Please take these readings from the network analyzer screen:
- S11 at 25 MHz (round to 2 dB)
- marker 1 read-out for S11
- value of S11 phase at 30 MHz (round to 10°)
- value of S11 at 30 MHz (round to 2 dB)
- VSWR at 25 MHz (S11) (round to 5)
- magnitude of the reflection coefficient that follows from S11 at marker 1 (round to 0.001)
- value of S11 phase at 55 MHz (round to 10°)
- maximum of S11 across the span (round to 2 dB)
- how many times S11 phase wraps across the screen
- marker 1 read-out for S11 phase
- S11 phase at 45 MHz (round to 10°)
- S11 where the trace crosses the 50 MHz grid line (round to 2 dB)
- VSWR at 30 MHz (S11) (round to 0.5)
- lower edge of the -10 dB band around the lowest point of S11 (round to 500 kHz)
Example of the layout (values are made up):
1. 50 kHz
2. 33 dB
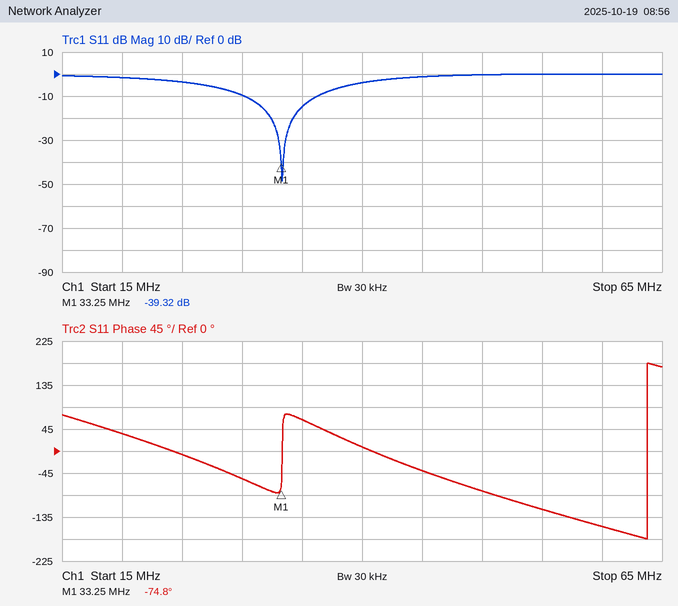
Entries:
1. -4 dB
2. -39.32 dB
3. -60°
4. -10 dB
5. 5
6. 0.011
7. -120°
8. 0 dB
9. 1
10. -74.8°
11. -40°
12. 0 dB
13. 2.0
14. 30.0 MHz
